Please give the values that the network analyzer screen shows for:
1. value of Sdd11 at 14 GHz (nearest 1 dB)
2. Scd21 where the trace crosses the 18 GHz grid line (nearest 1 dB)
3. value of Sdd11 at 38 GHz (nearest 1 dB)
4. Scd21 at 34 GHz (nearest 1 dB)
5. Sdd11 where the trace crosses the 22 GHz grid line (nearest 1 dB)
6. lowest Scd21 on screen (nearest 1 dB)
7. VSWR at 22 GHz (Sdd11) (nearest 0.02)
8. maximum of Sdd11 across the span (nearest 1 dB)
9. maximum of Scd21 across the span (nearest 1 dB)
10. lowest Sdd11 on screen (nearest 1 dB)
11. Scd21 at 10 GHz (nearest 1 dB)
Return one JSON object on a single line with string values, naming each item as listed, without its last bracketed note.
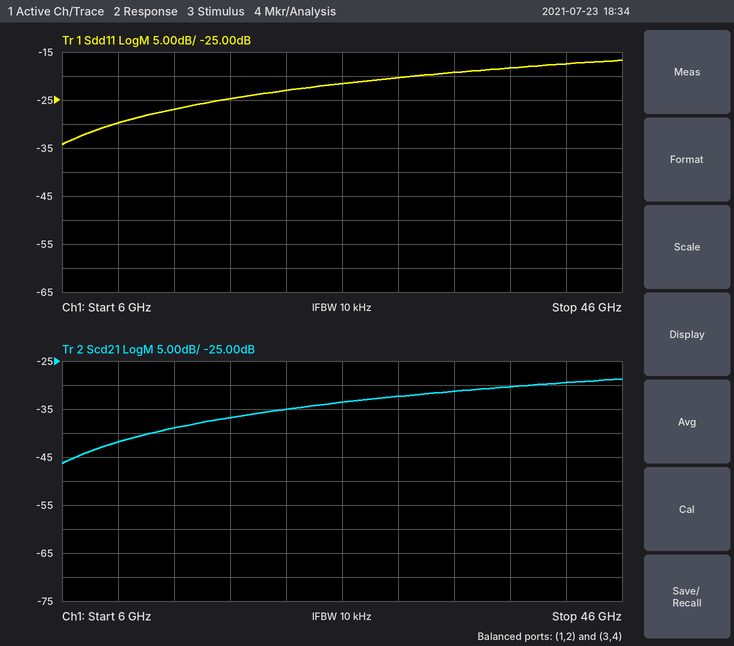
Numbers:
{"value of Sdd11 at 14 GHz": "-27 dB", "Scd21 where the trace crosses the 18 GHz grid line": "-37 dB", "value of Sdd11 at 38 GHz": "-18 dB", "Scd21 at 34 GHz": "-31 dB", "Sdd11 where the trace crosses the 22 GHz grid line": "-23 dB", "lowest Scd21 on screen": "-46 dB", "VSWR at 22 GHz (Sdd11)": "1.16", "maximum of Sdd11 across the span": "-17 dB", "maximum of Scd21 across the span": "-29 dB", "lowest Sdd11 on screen": "-34 dB", "Scd21 at 10 GHz": "-42 dB"}
